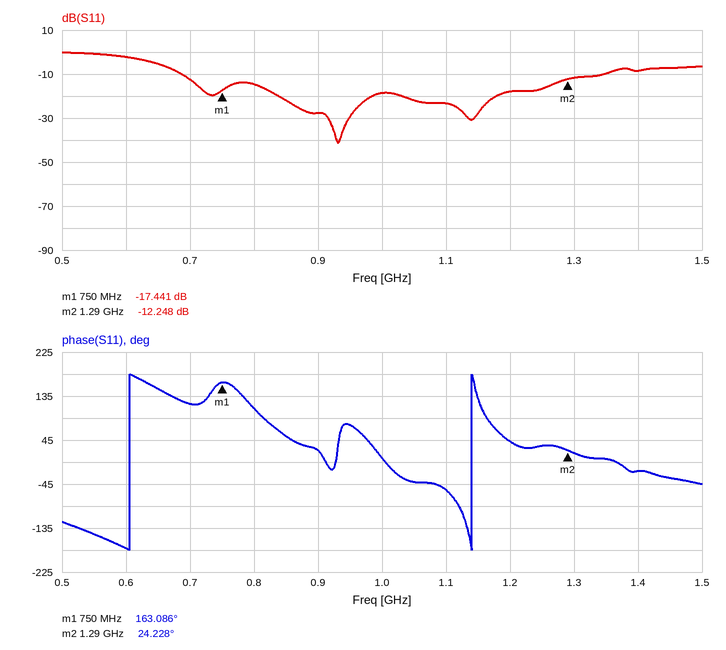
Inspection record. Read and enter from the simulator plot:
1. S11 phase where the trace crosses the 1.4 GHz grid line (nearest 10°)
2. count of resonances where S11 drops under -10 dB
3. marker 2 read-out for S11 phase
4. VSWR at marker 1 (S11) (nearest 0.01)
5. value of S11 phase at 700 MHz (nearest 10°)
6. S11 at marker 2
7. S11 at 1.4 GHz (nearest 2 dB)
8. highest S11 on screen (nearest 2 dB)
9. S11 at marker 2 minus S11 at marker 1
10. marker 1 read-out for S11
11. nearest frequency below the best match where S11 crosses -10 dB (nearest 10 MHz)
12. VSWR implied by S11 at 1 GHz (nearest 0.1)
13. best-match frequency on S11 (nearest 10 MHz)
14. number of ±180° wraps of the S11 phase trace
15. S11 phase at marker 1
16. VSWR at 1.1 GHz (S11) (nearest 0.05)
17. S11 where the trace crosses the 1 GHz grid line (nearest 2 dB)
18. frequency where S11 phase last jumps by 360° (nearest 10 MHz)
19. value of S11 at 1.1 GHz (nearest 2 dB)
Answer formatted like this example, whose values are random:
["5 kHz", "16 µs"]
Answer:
["-20°", "3", "24.228°", "1.31", "120°", "-12.248 dB", "-8 dB", "0 dB", "5.193 dB", "-17.441 dB", "690 MHz", "1.3", "930 MHz", "2", "163.086°", "1.15", "-18 dB", "1.14 GHz", "-24 dB"]
